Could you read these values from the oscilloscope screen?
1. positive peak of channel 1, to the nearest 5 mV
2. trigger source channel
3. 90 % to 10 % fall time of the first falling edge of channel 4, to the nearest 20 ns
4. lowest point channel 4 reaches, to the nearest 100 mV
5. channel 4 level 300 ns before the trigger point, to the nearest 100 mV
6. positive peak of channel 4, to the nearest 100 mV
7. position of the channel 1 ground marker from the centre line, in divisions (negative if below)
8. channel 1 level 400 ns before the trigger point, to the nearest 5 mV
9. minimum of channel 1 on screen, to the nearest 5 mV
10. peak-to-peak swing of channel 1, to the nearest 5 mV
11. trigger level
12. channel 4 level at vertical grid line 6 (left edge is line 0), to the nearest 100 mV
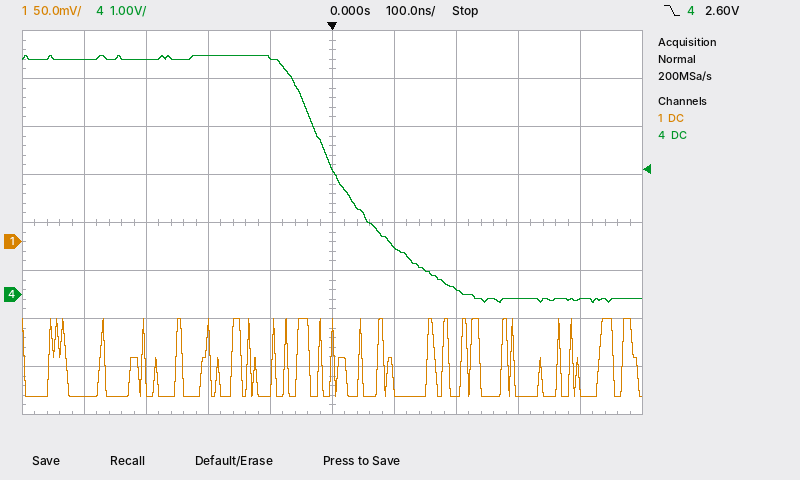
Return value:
-80 mV
channel 4
220 ns
-200 mV
4.9 V
5.0 V
-0.4 div
-160 mV
-160 mV
80 mV
2.60 V
1.0 V
